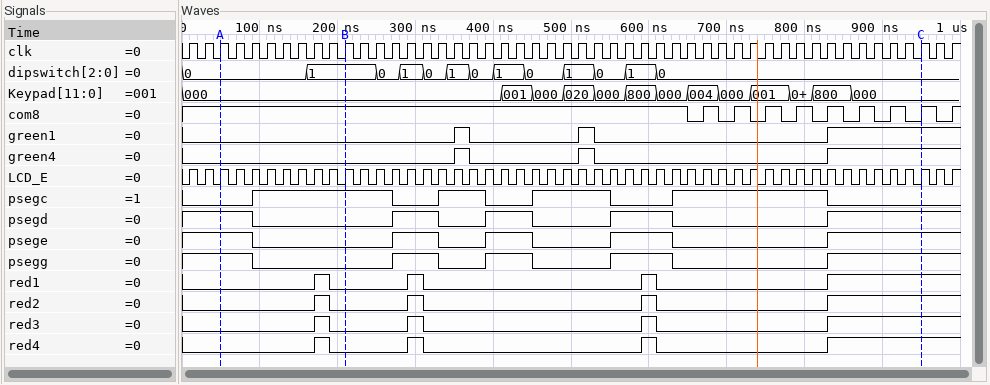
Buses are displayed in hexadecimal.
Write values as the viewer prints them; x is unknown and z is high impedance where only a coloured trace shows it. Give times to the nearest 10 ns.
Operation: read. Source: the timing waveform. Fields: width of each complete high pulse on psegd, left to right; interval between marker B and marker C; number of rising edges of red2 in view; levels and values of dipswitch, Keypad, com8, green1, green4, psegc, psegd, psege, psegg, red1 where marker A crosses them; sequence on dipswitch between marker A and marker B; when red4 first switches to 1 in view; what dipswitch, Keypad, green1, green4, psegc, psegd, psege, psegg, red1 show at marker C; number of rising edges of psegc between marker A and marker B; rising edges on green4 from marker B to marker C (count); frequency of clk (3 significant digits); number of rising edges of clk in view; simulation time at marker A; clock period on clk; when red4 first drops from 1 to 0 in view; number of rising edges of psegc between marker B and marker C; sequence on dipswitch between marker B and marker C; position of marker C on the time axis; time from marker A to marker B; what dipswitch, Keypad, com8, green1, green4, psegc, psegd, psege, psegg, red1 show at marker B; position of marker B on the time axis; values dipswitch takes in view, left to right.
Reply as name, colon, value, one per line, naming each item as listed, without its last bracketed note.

width of each complete high pulse on psegd, left to right: 60 ns, 60 ns, 80 ns
interval between marker B and marker C: 740 ns
number of rising edges of red2 in view: 4
levels and values of dipswitch, Keypad, com8, green1, green4, psegc, psegd, psege, psegg, red1 where marker A crosses them: dipswitch=0, Keypad=000, com8=1, green1=0, green4=0, psegc=0, psegd=1, psege=1, psegg=1, red1=0
sequence on dipswitch between marker A and marker B: 0, 1
when red4 first switches to 1 in view: 170 ns
what dipswitch, Keypad, green1, green4, psegc, psegd, psege, psegg, red1 show at marker C: dipswitch=0, Keypad=000, green1=1, green4=1, psegc=0, psegd=1, psege=1, psegg=1, red1=1
number of rising edges of psegc between marker A and marker B: 1
rising edges on green4 from marker B to marker C: 3
frequency of clk: 50.0 MHz
number of rising edges of clk in view: 50
simulation time at marker A: 50 ns
clock period on clk: 20 ns
when red4 first drops from 1 to 0 in view: 190 ns
number of rising edges of psegc between marker B and marker C: 3
sequence on dipswitch between marker B and marker C: 1, 0, 1, 0, 1, 0, 1, 0, 1, 0, 1, 0
position of marker C on the time axis: 950 ns
time from marker A to marker B: 160 ns
what dipswitch, Keypad, com8, green1, green4, psegc, psegd, psege, psegg, red1 show at marker B: dipswitch=1, Keypad=000, com8=1, green1=0, green4=0, psegc=1, psegd=0, psege=0, psegg=0, red1=0
position of marker B on the time axis: 210 ns
values dipswitch takes in view, left to right: 0, 1, 0, 1, 0, 1, 0, 1, 0, 1, 0, 1, 0
